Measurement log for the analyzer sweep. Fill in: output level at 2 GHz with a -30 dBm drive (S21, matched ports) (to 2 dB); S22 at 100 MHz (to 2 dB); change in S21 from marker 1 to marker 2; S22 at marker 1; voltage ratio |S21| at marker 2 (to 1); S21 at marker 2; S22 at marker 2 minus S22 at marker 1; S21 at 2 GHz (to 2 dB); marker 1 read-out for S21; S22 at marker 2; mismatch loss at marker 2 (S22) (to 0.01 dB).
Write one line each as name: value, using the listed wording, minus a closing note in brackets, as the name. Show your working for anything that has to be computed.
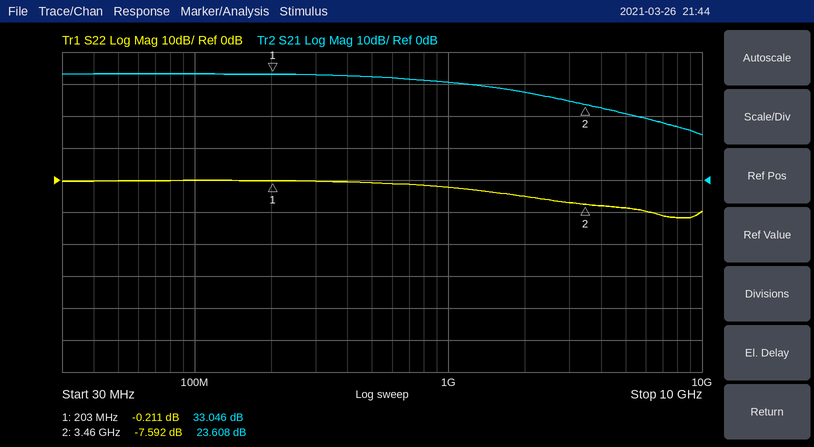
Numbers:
output level at 2 GHz with a -30 dBm drive (S21, matched ports): -30 dBm + (28 dB) = -2 dBm
S22 at 100 MHz: 0 dB
change in S21 from marker 1 to marker 2: 23.608 − (33.046) = -9.438 dB
S22 at marker 1: -0.211 dB
voltage ratio |S21| at marker 2: 10^(23.608/20) ≈ 15
S21 at marker 2: 23.608 dB
S22 at marker 2 minus S22 at marker 1: -7.592 − (-0.211) = -7.381 dB
S21 at 2 GHz: 28 dB
marker 1 read-out for S21: 33.046 dB
S22 at marker 2: -7.592 dB
mismatch loss at marker 2 (S22): −10 log10(1 − 10^(-7.592/10)) ≈ 0.83 dB
